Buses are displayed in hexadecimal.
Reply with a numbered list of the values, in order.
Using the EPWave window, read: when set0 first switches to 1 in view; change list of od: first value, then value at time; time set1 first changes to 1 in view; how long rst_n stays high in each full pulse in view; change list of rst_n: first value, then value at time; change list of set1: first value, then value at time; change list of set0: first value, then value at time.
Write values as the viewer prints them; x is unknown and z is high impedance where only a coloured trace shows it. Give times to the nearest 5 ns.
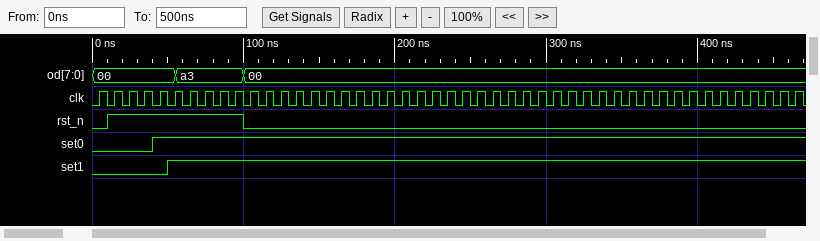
1. 40 ns
2. 00, a3 at 55 ns, 00 at 100 ns
3. 50 ns
4. 90 ns
5. 0, 1 at 10 ns, 0 at 100 ns
6. 0, 1 at 50 ns
7. 0, 1 at 40 ns
